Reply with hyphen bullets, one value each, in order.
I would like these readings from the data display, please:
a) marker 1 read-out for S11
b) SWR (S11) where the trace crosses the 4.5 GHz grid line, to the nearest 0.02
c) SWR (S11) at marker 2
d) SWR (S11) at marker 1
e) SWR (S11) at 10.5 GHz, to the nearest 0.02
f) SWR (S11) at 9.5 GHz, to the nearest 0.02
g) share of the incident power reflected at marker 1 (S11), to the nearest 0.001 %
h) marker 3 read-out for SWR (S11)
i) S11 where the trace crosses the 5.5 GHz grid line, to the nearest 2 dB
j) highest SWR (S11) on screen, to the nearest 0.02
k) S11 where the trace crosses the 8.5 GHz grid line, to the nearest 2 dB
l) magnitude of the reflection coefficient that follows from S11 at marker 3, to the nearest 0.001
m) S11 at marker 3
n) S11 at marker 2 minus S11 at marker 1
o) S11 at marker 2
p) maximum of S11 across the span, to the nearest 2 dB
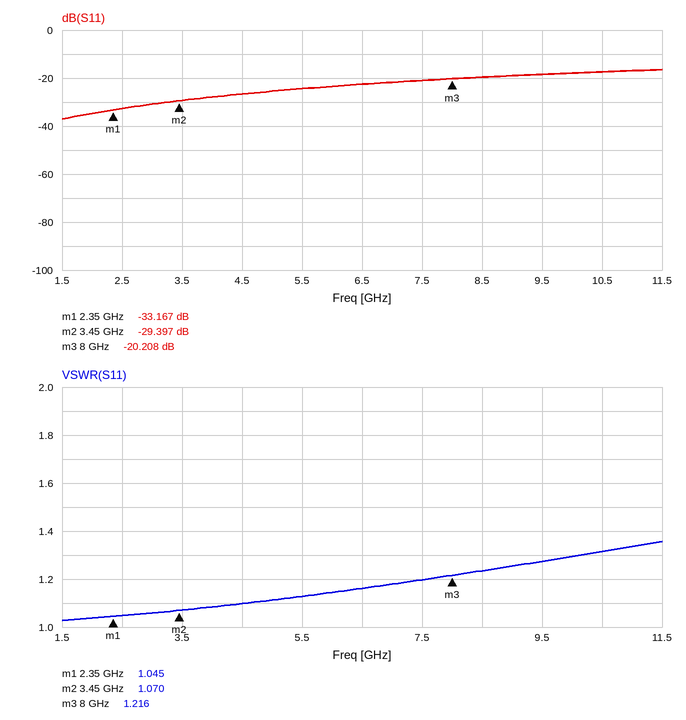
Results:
- -33.167 dB
- 1.10
- 1.070
- 1.045
- 1.32
- 1.28
- 0.048 %
- 1.216
- -24 dB
- 1.36
- -20 dB
- 0.098
- -20.208 dB
- 3.770 dB
- -29.397 dB
- -16 dB
